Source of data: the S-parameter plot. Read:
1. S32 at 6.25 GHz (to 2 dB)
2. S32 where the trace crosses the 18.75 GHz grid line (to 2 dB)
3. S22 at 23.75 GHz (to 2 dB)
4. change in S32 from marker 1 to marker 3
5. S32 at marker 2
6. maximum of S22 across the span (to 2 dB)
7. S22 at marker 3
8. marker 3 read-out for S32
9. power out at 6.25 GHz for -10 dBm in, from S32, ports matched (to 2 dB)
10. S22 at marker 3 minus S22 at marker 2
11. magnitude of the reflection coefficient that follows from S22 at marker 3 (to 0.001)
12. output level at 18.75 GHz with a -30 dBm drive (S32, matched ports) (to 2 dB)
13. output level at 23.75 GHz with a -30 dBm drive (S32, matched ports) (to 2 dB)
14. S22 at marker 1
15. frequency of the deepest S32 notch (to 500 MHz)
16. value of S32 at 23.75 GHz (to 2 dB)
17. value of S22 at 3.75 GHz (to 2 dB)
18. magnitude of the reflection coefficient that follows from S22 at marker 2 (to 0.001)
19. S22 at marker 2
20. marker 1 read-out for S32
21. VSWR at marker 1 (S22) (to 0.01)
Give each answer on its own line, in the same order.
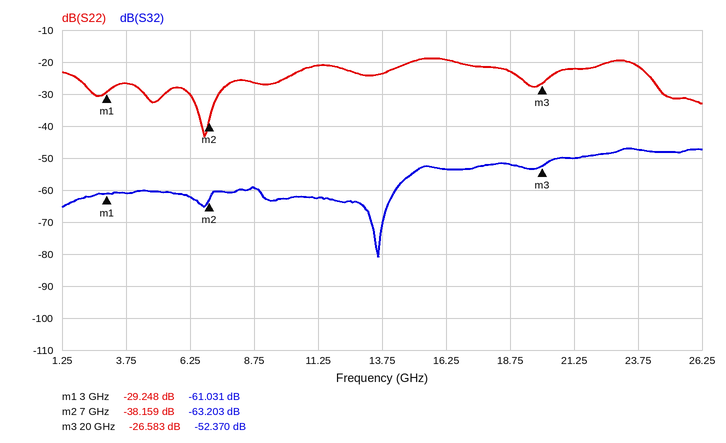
-62 dB
-52 dB
-22 dB
8.661 dB
-63.203 dB
-18 dB
-26.583 dB
-52.370 dB
-72 dBm
11.576 dB
0.047
-82 dBm
-78 dBm
-29.248 dB
13.5 GHz
-48 dB
-26 dB
0.012
-38.159 dB
-61.031 dB
1.07
